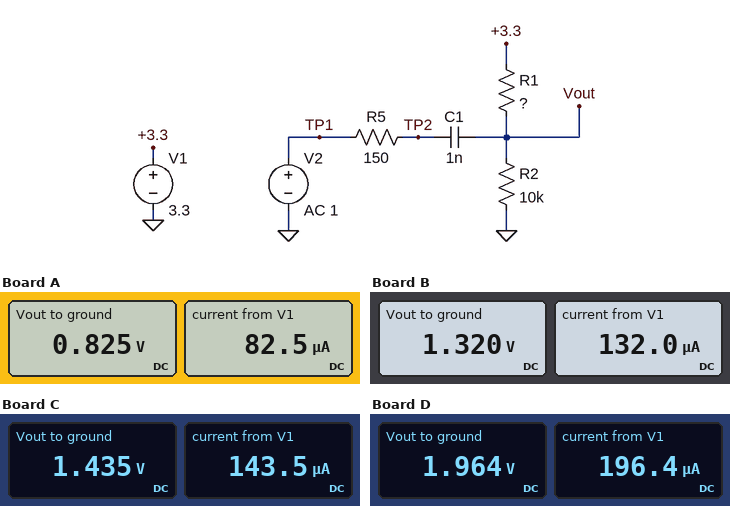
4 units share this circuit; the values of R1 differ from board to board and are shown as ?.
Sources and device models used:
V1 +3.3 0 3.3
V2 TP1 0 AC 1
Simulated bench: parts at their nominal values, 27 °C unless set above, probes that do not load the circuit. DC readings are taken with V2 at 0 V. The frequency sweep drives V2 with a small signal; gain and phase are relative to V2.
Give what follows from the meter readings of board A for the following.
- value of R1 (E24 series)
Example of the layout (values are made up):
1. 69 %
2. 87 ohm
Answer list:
1. 30 kΩ
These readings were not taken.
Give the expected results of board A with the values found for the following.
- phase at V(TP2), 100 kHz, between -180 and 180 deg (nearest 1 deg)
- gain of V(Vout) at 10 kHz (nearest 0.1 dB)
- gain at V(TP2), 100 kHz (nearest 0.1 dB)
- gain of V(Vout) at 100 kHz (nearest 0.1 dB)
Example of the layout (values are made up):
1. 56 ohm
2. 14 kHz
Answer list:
1. 0 deg
2. -7.4 dB
3. -0.2 dB
4. -0.4 dB
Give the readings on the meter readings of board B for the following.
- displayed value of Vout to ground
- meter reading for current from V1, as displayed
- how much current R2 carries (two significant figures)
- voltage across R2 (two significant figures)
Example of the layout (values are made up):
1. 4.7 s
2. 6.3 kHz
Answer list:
1. 1.320 V
2. 132.0 µA
3. 130 µA
4. 1.3 V
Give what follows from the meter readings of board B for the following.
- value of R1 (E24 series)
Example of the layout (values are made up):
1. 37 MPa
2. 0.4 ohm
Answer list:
1. 15 kΩ
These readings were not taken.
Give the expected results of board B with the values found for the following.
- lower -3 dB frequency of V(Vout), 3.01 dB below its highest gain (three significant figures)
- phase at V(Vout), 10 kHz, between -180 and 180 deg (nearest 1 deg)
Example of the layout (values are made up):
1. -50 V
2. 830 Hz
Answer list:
1. 25.9 kHz
2. 69 deg
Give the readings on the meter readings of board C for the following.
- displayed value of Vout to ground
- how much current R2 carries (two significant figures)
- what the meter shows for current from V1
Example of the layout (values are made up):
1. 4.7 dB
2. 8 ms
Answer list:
1. 1.435 V
2. 140 µA
3. 143.5 µA
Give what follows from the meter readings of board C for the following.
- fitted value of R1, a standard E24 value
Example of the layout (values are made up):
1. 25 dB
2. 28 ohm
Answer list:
1. 13 kΩ
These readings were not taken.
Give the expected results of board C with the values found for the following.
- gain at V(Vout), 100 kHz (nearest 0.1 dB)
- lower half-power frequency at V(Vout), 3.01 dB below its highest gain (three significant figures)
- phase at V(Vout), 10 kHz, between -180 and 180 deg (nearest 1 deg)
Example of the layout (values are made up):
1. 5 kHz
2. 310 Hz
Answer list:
1. -0.5 dB
2. 27.4 kHz
3. 70 deg
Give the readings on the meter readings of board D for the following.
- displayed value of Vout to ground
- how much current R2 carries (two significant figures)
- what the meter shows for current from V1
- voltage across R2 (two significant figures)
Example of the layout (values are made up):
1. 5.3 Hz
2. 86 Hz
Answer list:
1. 1.964 V
2. 200 µA
3. 196.4 µA
4. 2.0 V
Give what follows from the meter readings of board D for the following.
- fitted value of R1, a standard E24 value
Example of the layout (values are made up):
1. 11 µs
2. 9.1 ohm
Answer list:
1. 6.8 kΩ
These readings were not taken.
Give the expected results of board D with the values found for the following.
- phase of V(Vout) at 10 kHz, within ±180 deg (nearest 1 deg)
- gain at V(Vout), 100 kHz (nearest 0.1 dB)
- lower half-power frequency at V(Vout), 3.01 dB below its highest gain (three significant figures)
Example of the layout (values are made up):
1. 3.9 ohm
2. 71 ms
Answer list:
1. 75 deg
2. -0.9 dB
3. 37.9 kHz
